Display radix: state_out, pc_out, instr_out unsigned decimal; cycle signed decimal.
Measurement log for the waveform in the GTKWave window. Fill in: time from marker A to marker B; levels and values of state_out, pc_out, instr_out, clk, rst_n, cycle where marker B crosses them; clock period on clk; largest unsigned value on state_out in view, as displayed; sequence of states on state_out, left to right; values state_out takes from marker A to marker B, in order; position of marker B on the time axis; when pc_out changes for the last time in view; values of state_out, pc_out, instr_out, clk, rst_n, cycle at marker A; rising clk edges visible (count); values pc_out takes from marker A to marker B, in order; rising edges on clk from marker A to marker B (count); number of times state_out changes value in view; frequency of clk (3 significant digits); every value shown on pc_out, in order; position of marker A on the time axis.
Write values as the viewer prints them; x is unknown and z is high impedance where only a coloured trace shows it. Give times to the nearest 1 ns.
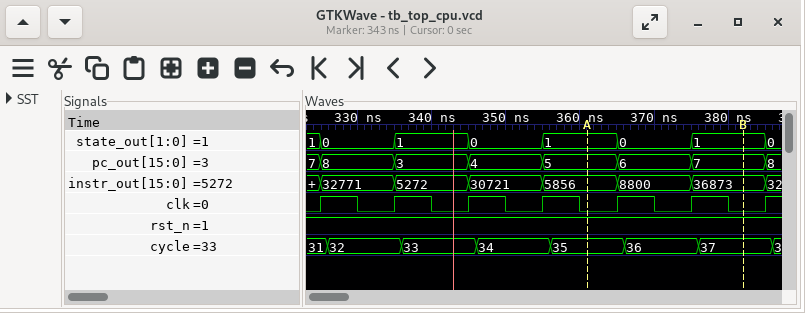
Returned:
21 ns
state_out=1, pc_out=7, instr_out=36873, clk=0, rst_n=1, cycle=37
10 ns
1
1, 0, 1, 0, 1, 0, 1, 0
1, 0, 1
382 ns
385 ns
state_out=1, pc_out=5, instr_out=5856, clk=0, rst_n=1, cycle=35
7
5, 6, 7
2
7
100 MHz
7, 8, 3, 4, 5, 6, 7, 8
361 ns
